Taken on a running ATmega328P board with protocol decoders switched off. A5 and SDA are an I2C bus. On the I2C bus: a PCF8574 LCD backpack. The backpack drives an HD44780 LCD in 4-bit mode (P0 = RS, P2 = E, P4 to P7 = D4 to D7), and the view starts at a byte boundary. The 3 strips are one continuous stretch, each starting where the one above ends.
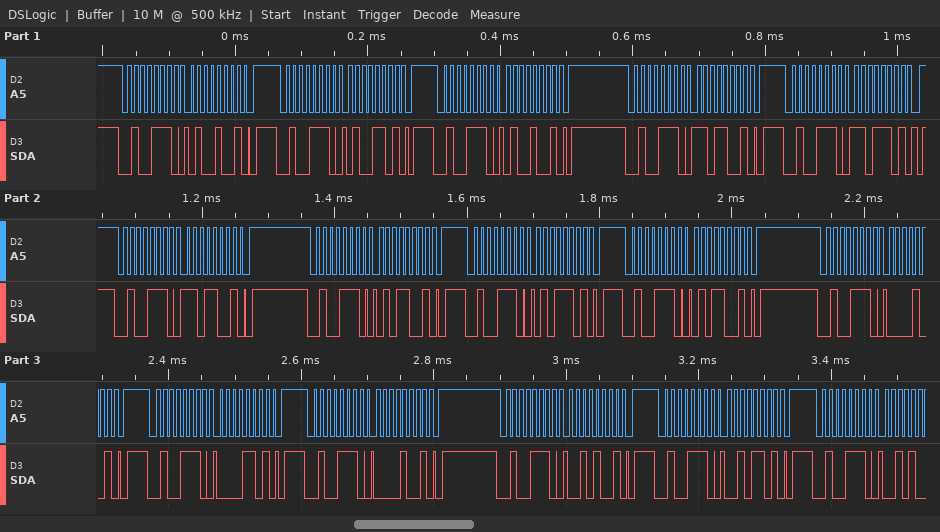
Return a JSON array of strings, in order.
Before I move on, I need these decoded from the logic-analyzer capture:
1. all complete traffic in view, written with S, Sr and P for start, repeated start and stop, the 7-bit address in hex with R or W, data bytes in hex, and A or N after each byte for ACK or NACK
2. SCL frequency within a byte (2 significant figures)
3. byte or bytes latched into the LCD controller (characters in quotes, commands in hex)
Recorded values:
["S 27W A 49 A P S 27W A 4D A P S 27W A 49 A P S 27W A D9 A P S 27W A DD A P S 27W A D9 A P S 27W A 59 A P S 27W A 5D A P S 27W A 59 A P S 27W A 09 A P S 27W A 0D A P S 27W A 09 A P S 27W A 29 A P S 27W A 2D A P S 27W A", "100 kHz", "'M' 'P'"]
